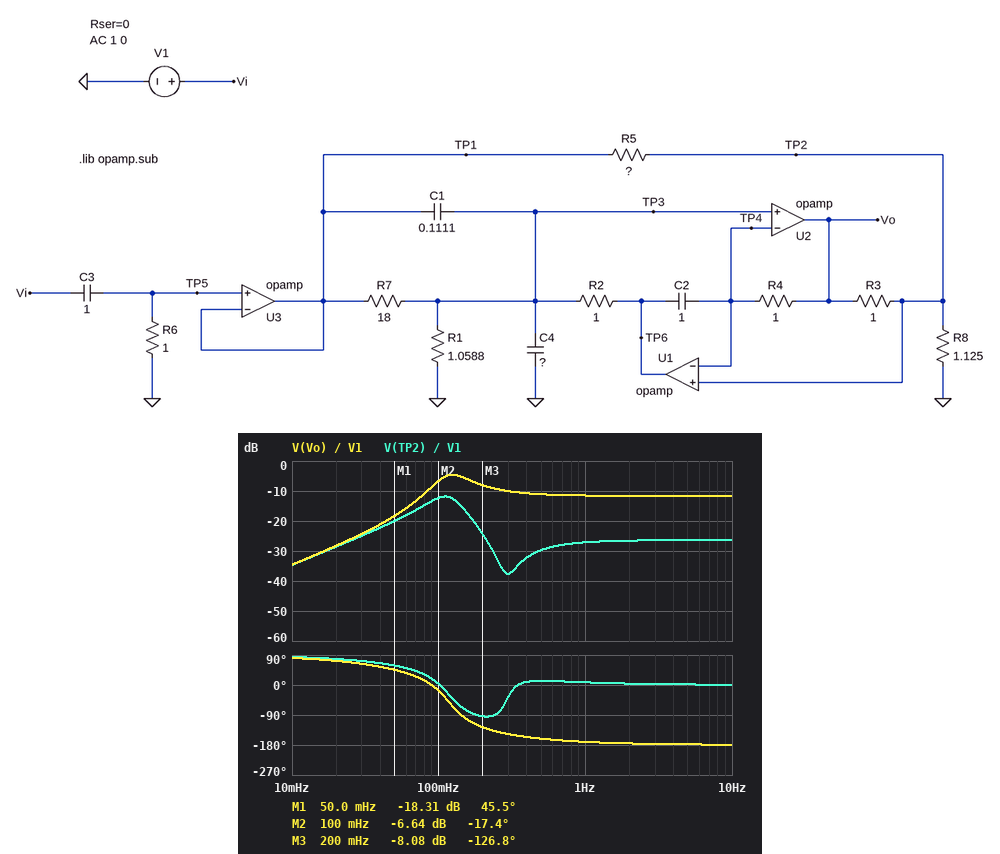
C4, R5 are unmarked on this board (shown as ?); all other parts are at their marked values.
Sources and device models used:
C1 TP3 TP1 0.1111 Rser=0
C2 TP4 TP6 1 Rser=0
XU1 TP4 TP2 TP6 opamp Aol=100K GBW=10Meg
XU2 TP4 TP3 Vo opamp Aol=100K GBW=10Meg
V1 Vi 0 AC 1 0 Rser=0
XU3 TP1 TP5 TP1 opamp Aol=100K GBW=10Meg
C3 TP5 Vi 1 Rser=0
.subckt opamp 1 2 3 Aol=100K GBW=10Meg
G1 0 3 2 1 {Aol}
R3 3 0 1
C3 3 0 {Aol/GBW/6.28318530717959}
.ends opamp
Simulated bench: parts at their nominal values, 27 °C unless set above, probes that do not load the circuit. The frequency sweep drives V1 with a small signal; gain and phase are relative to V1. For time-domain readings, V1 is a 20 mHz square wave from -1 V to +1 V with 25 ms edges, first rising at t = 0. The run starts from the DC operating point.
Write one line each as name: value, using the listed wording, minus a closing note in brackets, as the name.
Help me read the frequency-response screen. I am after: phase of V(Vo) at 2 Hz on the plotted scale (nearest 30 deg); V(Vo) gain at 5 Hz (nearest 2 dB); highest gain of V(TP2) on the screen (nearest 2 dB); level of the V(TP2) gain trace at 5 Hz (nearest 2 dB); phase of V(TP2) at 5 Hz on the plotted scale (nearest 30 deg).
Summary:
phase of V(Vo) at 2 Hz on the plotted scale: -180 deg
V(Vo) gain at 5 Hz: -12 dB
highest gain of V(TP2) on the screen: -12 dB
level of the V(TP2) gain trace at 5 Hz: -26 dB
phase of V(TP2) at 5 Hz on the plotted scale: 0 deg
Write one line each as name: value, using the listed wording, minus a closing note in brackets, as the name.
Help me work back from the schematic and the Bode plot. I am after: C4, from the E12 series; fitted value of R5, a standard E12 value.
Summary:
C4, from the E12 series: 2.2 F
fitted value of R5, a standard E12 value: 2.7 Ω
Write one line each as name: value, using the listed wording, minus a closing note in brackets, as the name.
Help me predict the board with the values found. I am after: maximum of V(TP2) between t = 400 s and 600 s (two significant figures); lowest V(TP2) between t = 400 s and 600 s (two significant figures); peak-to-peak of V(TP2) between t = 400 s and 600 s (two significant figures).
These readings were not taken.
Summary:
maximum of V(TP2) between t = 400 s and 600 s: 210 mV
lowest V(TP2) between t = 400 s and 600 s: -210 mV
peak-to-peak of V(TP2) between t = 400 s and 600 s: 420 mV
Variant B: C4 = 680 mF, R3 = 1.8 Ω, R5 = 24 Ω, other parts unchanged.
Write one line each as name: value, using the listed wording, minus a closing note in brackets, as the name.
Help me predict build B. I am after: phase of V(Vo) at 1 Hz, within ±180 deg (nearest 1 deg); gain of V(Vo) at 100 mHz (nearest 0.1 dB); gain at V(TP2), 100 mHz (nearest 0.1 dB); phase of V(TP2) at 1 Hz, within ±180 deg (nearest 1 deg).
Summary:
phase of V(Vo) at 1 Hz, within ±180 deg: 18 deg
gain of V(Vo) at 100 mHz: -35.0 dB
gain at V(TP2), 100 mHz: -35.6 dB
phase of V(TP2) at 1 Hz, within ±180 deg: 16 deg
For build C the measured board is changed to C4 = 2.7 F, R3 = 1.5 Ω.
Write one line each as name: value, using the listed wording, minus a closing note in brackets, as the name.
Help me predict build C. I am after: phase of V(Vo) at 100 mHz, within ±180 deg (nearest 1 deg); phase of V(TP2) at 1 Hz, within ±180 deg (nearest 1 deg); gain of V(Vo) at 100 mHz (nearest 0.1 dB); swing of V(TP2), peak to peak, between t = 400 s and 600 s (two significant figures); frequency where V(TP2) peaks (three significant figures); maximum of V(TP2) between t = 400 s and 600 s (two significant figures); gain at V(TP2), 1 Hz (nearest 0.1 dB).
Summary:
phase of V(Vo) at 100 mHz, within ±180 deg: 6 deg
phase of V(TP2) at 1 Hz, within ±180 deg: 7 deg
gain of V(Vo) at 100 mHz: -4.9 dB
swing of V(TP2), peak to peak, between t = 400 s and 600 s: 500 mV
frequency where V(TP2) peaks: 126 mHz
maximum of V(TP2) between t = 400 s and 600 s: 250 mV
gain at V(TP2), 1 Hz: -29.2 dB
